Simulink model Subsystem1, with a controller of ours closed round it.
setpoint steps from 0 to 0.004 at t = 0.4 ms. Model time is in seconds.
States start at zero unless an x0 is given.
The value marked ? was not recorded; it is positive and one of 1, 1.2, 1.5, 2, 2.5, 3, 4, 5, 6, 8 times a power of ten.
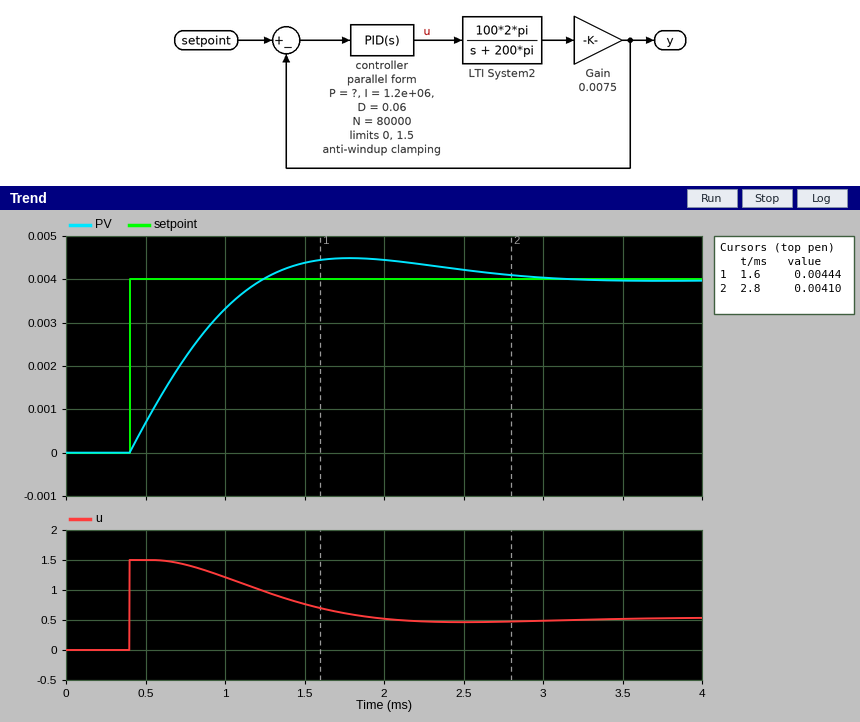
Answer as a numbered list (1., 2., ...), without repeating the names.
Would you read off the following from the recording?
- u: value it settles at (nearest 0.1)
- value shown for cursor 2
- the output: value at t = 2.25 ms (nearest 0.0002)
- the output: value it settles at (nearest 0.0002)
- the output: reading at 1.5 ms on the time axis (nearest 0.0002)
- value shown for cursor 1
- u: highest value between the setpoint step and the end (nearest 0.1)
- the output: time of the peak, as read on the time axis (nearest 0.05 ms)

1. 0.5
2. 0.00410
3. 0.0044
4. 0.0040
5. 0.0044
6. 0.00444
7. 1.5
8. 1.80 ms
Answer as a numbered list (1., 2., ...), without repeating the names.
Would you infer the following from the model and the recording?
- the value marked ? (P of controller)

1. 600
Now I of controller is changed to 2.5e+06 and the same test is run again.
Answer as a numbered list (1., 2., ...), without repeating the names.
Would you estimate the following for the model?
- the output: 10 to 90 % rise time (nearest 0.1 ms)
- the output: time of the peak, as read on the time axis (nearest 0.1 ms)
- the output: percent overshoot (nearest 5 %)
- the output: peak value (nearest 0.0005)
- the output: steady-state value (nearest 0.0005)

1. 0.6 ms
2. 1.5 ms
3. 15 %
4. 0.0045
5. 0.0040
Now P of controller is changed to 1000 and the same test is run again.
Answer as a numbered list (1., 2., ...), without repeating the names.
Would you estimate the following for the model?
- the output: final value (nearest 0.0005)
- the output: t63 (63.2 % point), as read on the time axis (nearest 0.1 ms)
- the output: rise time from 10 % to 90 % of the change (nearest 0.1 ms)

1. 0.0040
2. 0.8 ms
3. 0.7 ms
